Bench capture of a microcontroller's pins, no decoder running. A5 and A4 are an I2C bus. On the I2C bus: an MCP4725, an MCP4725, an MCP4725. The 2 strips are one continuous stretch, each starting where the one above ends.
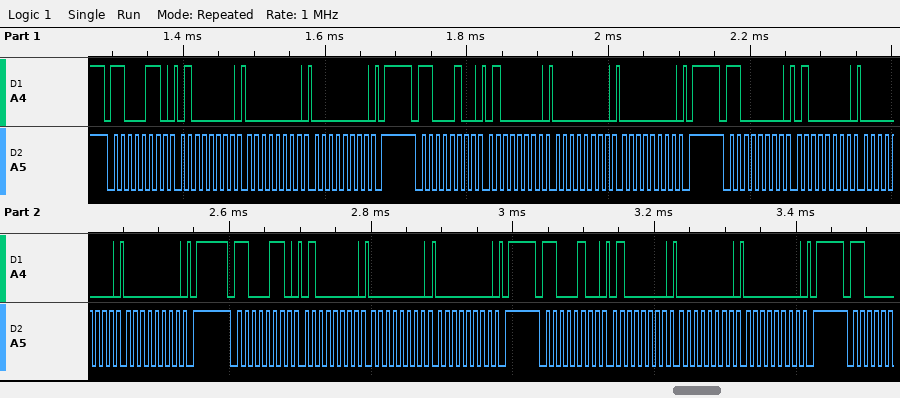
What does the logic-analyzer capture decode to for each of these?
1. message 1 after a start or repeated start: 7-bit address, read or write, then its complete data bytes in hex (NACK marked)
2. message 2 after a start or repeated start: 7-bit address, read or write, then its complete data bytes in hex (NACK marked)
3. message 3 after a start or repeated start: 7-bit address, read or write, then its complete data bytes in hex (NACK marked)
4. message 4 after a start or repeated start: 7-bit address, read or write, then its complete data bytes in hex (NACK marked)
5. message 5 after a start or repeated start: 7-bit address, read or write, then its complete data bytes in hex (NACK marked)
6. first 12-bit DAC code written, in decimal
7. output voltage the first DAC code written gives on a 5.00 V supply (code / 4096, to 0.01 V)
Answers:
0x63 write: 40 00 00
0x62 write: 40 00 00
0x60 write: 40 00 00
0x63 write: 40 00 00
0x62 write: 40 00 00
0
0.00 V
